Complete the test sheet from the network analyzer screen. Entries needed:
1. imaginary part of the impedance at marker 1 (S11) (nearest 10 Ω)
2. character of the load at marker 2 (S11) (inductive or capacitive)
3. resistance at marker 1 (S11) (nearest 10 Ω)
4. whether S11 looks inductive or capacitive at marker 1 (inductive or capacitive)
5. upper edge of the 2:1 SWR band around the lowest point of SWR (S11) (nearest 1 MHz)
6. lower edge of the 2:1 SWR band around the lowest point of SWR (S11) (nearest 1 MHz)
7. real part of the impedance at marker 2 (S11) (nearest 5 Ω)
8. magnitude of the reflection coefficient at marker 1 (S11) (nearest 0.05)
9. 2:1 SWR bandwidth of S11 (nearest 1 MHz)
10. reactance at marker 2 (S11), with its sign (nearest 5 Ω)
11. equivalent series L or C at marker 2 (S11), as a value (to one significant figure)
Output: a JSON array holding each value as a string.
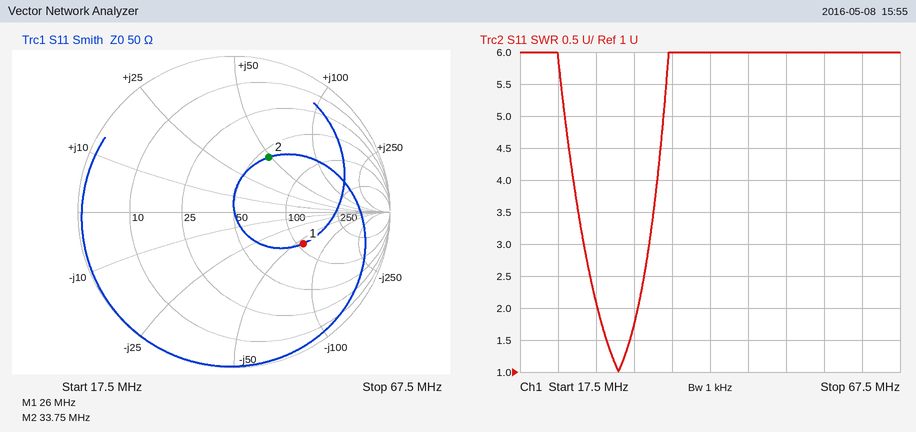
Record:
["-60 Ω", "inductive", "110 Ω", "capacitive", "33 MHz", "28 MHz", "55 Ω", "0.50", "5 MHz", "+50 Ω", "200 nH"]
